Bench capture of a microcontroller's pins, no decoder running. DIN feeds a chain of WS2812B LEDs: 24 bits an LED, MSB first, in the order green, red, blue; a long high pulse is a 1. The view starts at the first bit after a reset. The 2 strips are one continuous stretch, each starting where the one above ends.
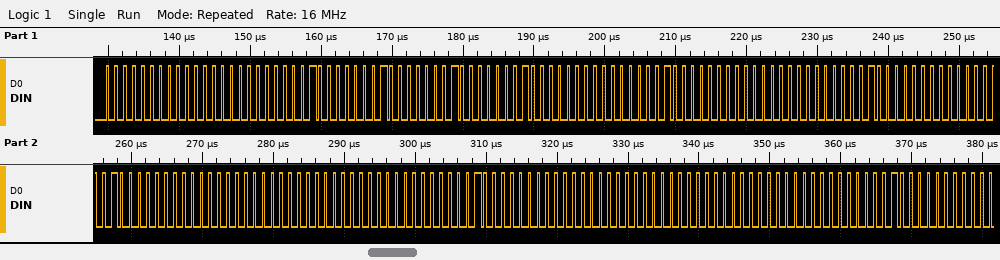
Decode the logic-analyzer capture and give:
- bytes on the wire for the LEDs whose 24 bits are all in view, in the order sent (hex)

00 00 01 01 01 01 00 01 00 00 02 00 02 00 00 00 00 01 00 00 00 00 00 02
